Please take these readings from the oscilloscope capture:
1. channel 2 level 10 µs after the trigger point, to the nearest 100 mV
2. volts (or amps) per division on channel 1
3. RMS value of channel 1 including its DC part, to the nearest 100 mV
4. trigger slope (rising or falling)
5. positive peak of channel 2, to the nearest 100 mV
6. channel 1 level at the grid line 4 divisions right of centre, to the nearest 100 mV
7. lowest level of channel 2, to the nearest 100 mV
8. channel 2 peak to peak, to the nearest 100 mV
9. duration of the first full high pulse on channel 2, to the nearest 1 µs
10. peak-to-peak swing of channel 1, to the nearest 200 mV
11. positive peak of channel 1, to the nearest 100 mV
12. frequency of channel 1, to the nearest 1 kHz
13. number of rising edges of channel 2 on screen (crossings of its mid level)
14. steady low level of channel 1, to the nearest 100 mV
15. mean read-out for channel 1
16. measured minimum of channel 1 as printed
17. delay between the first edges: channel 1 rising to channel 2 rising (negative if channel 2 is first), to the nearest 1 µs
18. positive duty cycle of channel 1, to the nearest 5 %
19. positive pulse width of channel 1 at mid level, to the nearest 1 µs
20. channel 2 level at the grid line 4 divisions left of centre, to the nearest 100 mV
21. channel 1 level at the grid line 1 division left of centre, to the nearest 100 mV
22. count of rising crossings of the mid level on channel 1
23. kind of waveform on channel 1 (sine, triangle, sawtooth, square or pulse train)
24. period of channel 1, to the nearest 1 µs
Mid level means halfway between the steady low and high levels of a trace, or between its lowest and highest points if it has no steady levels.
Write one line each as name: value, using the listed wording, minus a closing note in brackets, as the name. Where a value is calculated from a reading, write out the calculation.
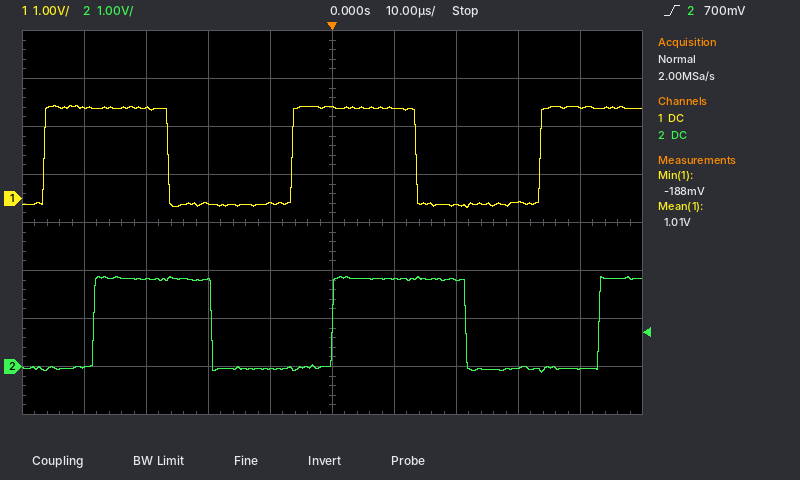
channel 2 level 10 µs after the trigger point, to the nearest 100 mV: 1.8 V
volts (or amps) per division on channel 1: 1 V
RMS value of channel 1 including its DC part, to the nearest 100 mV: √(0.5 × (1.9 V)² + 0.5 × (-100 mV)²) ≈ 1.3 V
trigger slope: rising
positive peak of channel 2, to the nearest 100 mV: 1.9 V
channel 1 level at the grid line 4 divisions right of centre, to the nearest 100 mV: 1.9 V
lowest level of channel 2, to the nearest 100 mV: -100 mV
channel 2 peak to peak, to the nearest 100 mV: 1.9 V − (-100 mV) = 2.0 V
duration of the first full high pulse on channel 2, to the nearest 1 µs: 19 µs
peak-to-peak swing of channel 1, to the nearest 200 mV: 2.2 V
positive peak of channel 1, to the nearest 100 mV: 1.9 V
frequency of channel 1, to the nearest 1 kHz: 1 / 40 µs ≈ 25 kHz
number of rising edges of channel 2 on screen: 3
steady low level of channel 1, to the nearest 100 mV: -100 mV
mean read-out for channel 1: 1.01 V
measured minimum of channel 1 as printed: -188 mV
delay between the first edges: channel 1 rising to channel 2 rising (negative if channel 2 is first), to the nearest 1 µs: +8 µs
positive duty cycle of channel 1, to the nearest 5 %: 20 µs / 40 µs ≈ 50 %
positive pulse width of channel 1 at mid level, to the nearest 1 µs: 20 µs
channel 2 level at the grid line 4 divisions left of centre, to the nearest 100 mV: 0.0 V
channel 1 level at the grid line 1 division left of centre, to the nearest 100 mV: -100 mV
count of rising crossings of the mid level on channel 1: 3
kind of waveform on channel 1: square
period of channel 1, to the nearest 1 µs: 40 µs
